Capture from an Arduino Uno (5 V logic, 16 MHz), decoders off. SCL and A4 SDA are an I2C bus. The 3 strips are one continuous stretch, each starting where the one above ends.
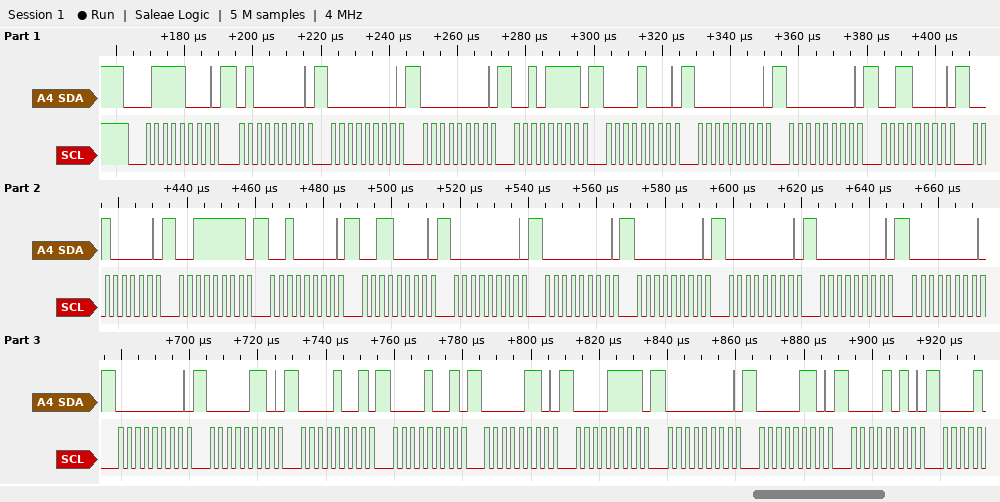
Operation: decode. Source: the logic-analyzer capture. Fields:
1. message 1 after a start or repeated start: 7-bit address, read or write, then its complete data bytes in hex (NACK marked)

0x3C write: 40 00 00 2F 08 00 00 30 20 3F 20 30 00 00 00 00 00 00 00 06 09 09 06 0F 00 06 0A
